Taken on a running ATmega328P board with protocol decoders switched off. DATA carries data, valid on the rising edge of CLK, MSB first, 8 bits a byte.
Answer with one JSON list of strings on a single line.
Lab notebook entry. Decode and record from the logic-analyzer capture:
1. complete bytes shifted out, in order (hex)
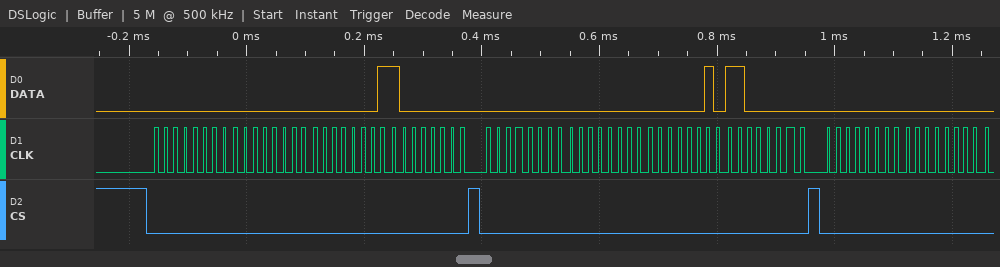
["0x00 0x00 0x01 0x80 0x00 0x00 0x02 0xC0 0x00 0x00"]
